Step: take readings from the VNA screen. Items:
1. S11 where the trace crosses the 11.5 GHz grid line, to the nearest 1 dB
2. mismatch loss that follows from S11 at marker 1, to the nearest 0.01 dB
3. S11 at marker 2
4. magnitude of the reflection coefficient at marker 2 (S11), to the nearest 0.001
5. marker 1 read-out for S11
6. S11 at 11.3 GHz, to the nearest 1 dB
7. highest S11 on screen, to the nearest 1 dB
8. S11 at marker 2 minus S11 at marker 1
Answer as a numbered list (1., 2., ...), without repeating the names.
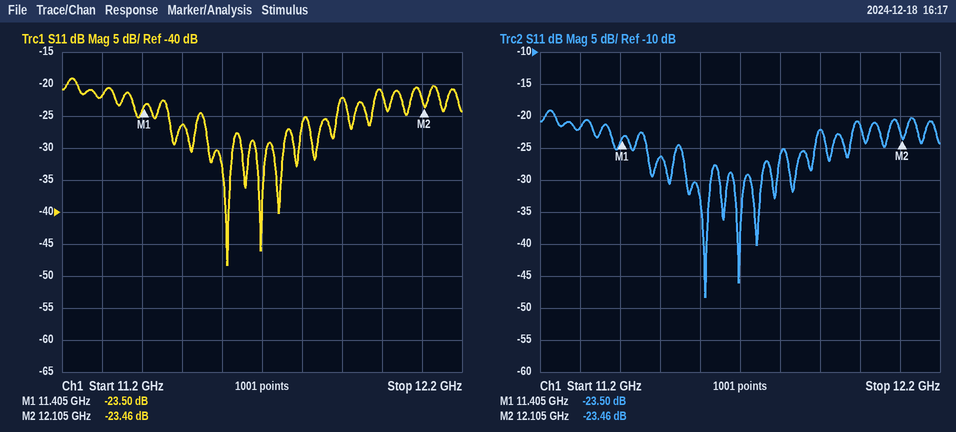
1. -26 dB
2. 0.02 dB
3. -23.46 dB
4. 0.067
5. -23.50 dB
6. -22 dB
7. -19 dB
8. 0.04 dB
